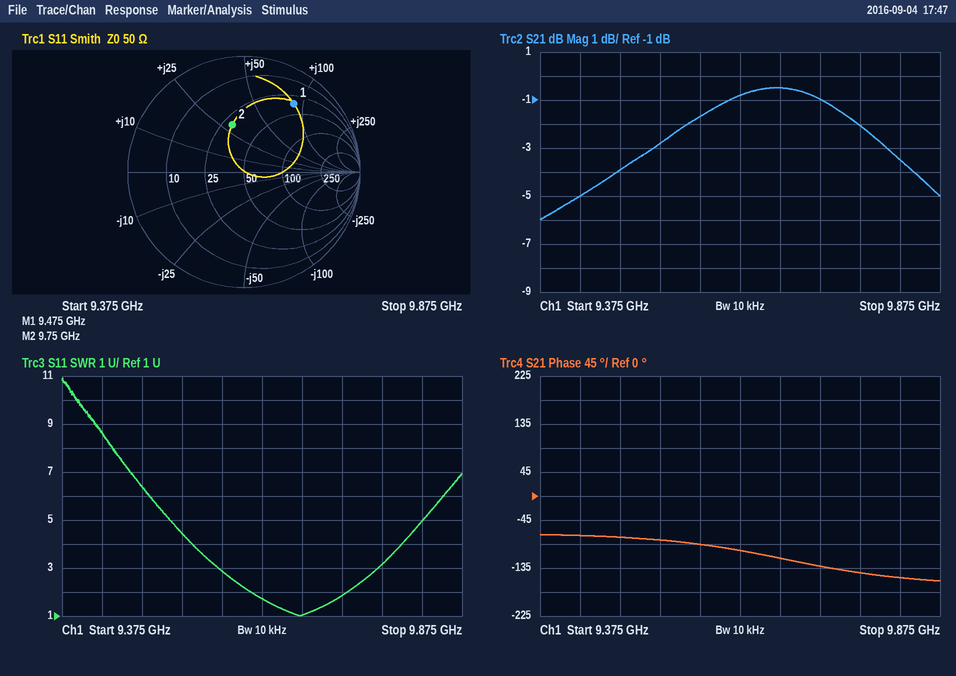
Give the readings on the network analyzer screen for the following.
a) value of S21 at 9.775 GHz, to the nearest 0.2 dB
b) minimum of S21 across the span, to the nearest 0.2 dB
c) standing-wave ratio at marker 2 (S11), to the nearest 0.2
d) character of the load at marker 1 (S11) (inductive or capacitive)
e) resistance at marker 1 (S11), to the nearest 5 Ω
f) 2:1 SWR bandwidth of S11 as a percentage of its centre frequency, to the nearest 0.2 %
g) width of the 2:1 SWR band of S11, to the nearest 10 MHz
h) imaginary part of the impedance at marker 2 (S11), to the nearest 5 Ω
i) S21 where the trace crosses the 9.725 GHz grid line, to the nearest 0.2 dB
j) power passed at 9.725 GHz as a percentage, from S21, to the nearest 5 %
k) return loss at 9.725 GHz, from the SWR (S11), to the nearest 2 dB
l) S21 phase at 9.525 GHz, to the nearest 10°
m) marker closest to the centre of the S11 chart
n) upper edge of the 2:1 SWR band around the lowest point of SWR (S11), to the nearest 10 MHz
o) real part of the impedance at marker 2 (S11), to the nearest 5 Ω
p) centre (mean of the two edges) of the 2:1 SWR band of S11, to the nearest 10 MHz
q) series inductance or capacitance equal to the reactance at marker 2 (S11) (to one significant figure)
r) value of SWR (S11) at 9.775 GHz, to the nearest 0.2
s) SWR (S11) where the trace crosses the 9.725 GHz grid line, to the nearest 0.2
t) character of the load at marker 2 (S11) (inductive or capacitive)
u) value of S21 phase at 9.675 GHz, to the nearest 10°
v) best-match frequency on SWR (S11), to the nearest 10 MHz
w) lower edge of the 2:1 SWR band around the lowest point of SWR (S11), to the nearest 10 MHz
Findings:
-2.0 dB
-6.0 dB
2.4
inductive
35 Ω
1.2 %
120 MHz
+30 Ω
-1.0 dB
80 %
10 dB
-80°
marker 2
9.73 GHz
30 Ω
9.67 GHz
500 pH
3.2
1.8
inductive
-120°
9.67 GHz
9.61 GHz
